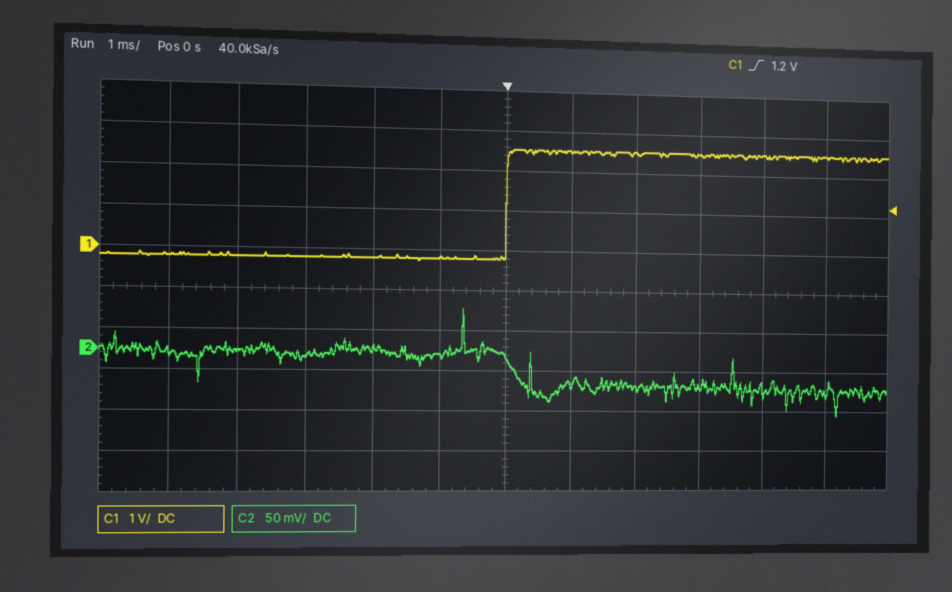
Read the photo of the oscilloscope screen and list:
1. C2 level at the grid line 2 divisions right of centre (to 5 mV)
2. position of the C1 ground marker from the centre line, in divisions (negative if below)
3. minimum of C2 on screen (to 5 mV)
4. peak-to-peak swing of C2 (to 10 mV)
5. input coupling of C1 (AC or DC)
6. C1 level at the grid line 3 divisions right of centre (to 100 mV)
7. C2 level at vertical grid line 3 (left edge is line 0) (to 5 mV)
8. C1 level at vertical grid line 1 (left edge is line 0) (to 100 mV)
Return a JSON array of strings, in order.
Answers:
["-45 mV", "+1.0 div", "-80 mV", "130 mV", "DC", "2.5 V", "-5 mV", "-200 mV"]
